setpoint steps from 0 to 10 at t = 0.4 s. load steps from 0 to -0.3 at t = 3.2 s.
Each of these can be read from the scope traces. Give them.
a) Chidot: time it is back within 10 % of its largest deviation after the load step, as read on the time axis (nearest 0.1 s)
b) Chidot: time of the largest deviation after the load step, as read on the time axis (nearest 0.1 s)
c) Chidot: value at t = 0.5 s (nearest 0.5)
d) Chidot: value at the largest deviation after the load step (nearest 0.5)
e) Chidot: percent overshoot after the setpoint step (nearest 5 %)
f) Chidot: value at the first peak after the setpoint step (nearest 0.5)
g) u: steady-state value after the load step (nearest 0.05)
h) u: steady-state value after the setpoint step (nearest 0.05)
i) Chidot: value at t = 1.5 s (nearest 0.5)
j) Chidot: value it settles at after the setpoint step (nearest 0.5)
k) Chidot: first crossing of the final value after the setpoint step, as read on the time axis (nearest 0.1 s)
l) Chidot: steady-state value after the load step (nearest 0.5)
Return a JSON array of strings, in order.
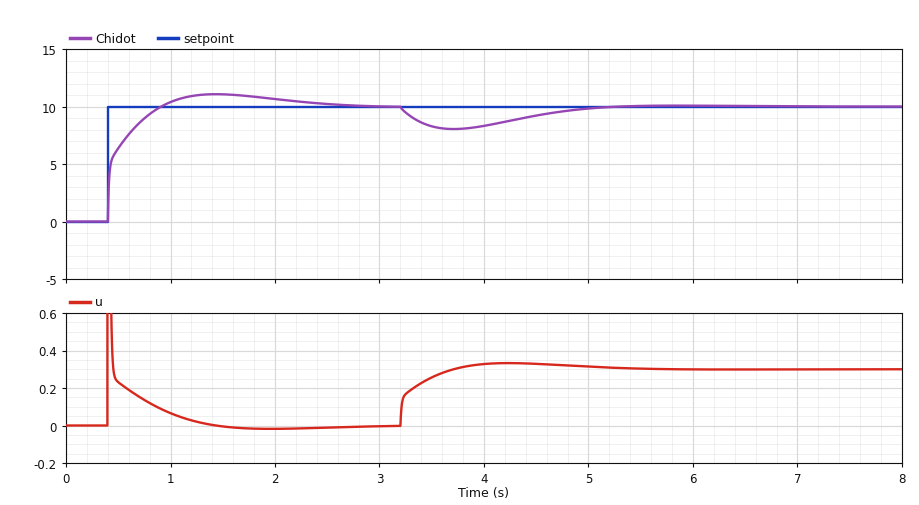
["5.0 s", "3.7 s", "6.5", "8.0", "10 %", "11.0", "0.30", "0.00", "11.0", "10.0", "0.9 s", "10.0"]
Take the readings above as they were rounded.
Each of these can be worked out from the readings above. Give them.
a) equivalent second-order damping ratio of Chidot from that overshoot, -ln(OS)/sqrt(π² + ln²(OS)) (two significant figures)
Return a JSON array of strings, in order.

["0.59"]
